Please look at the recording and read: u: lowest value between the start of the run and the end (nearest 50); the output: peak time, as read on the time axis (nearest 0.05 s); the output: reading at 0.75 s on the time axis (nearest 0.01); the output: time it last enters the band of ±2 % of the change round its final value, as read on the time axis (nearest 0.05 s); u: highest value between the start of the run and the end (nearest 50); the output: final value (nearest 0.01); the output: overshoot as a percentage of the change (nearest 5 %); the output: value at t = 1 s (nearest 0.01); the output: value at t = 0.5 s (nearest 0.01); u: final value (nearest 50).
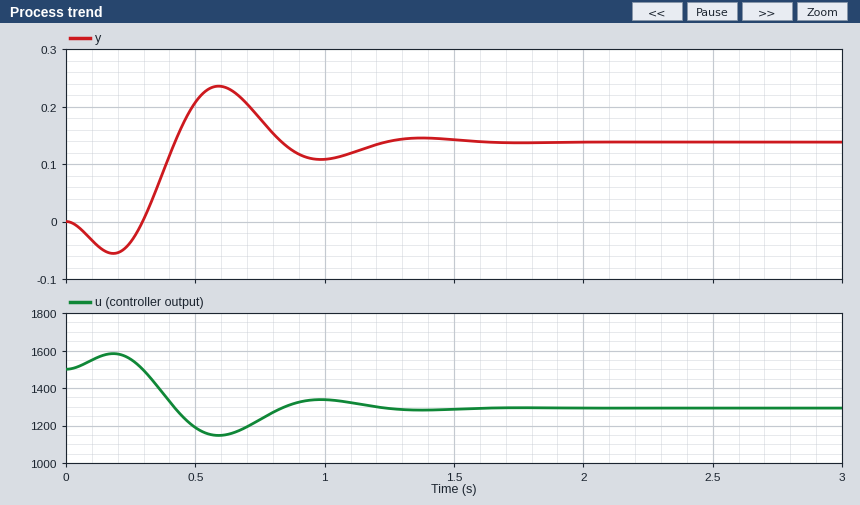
1150
0.60 s
0.18
1.55 s
1600
0.14
70 %
0.11
0.21
1300
